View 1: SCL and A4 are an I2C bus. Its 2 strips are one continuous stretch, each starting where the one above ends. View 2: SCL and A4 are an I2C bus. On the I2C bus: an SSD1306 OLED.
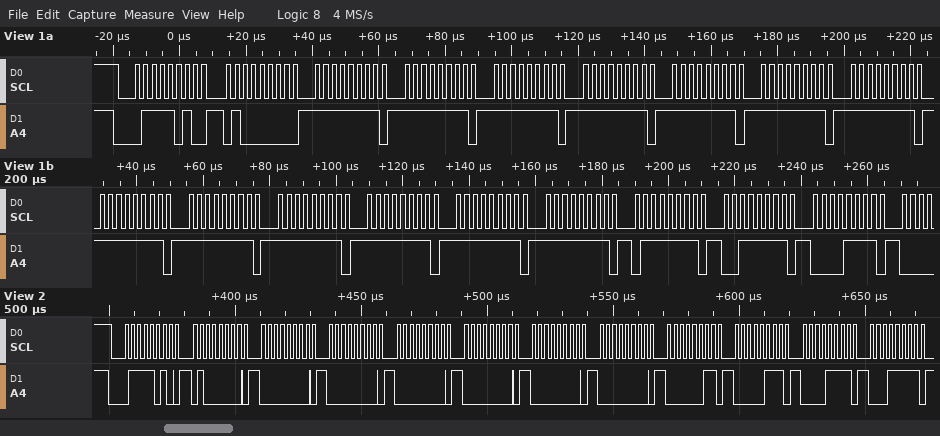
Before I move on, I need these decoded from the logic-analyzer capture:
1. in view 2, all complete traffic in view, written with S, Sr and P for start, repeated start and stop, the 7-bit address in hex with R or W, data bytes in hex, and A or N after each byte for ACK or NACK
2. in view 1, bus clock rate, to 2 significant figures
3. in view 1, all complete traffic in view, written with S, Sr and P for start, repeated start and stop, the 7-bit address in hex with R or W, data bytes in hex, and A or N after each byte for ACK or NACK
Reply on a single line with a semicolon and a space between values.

S 3DW A 40 A 00 A 00 A 00 A 00 A 00 A 00 A 03 A 07 A 0F A 1F A; 400 kHz; S 3DW A 40 A FF A FF A FF A FF A FF A FF A FF A FF A FF A FF A FF A FF A FF A 7F A 3F A 0F A
